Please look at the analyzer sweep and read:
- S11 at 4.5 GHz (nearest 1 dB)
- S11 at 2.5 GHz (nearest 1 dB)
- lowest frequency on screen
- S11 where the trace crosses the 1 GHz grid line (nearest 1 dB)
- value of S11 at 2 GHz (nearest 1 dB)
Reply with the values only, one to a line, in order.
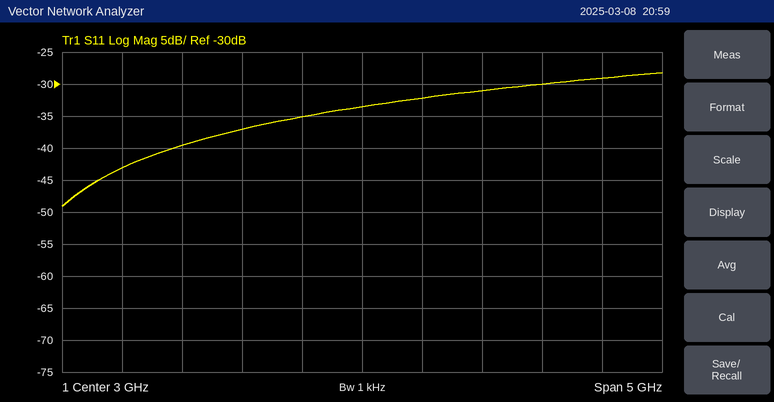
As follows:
-30 dB
-35 dB
500 MHz
-43 dB
-37 dB
